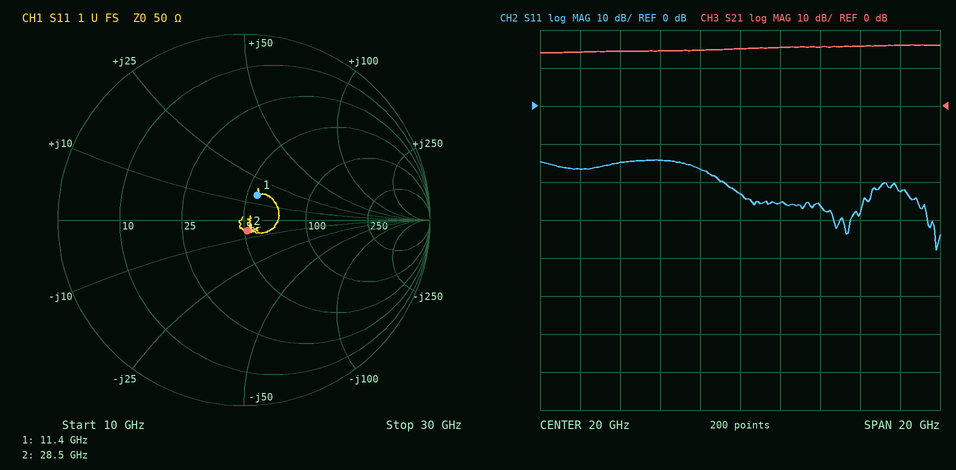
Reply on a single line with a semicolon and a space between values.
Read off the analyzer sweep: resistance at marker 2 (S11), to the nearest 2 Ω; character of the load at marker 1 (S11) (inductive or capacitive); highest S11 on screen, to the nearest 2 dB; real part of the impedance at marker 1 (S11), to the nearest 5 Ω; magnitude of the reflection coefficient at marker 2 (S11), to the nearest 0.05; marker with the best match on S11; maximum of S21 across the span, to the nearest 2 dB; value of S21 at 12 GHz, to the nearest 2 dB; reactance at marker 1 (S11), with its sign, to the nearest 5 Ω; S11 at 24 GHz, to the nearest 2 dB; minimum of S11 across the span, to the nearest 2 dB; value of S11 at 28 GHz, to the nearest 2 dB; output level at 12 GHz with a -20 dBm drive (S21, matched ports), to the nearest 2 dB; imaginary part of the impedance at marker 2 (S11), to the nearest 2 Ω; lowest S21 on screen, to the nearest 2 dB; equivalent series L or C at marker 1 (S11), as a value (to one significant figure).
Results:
52 Ω; inductive; -14 dB; 55 Ω; 0.05; marker 2; 16 dB; 14 dB; +15 Ω; -26 dB; -38 dB; -22 dB; -6 dBm; -6 Ω; 14 dB; 200 pH
